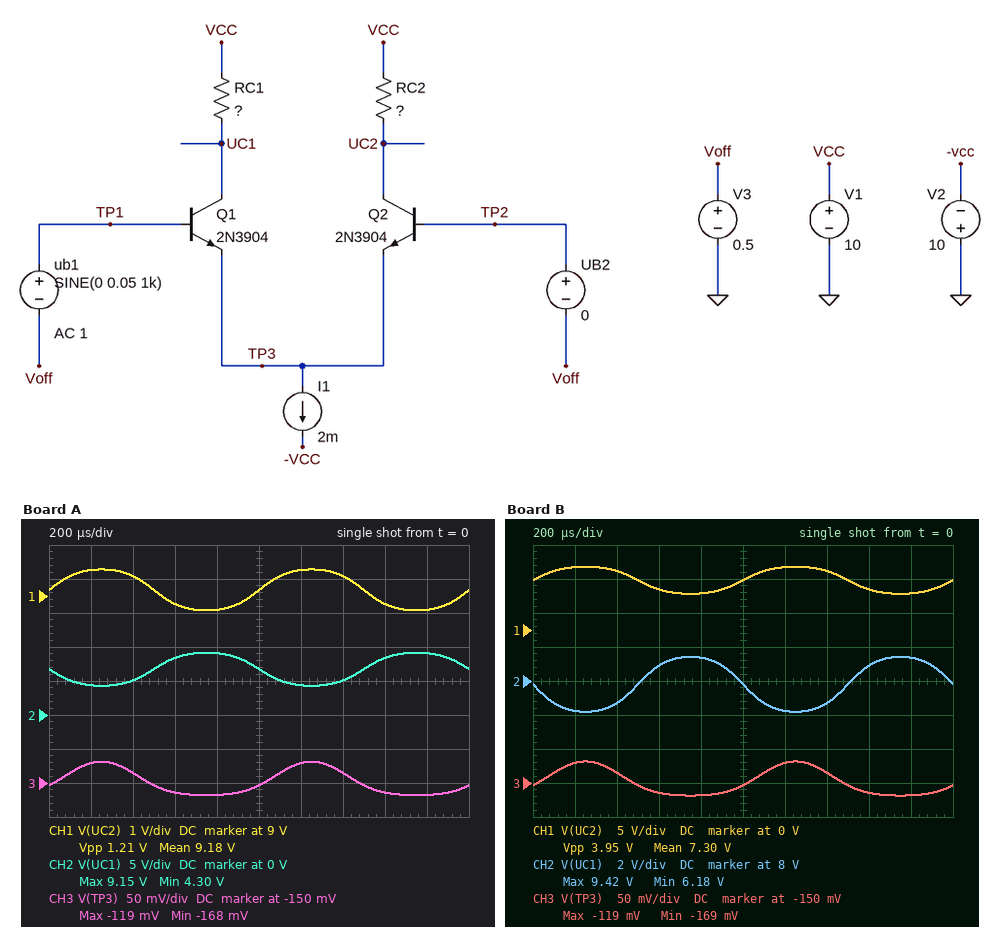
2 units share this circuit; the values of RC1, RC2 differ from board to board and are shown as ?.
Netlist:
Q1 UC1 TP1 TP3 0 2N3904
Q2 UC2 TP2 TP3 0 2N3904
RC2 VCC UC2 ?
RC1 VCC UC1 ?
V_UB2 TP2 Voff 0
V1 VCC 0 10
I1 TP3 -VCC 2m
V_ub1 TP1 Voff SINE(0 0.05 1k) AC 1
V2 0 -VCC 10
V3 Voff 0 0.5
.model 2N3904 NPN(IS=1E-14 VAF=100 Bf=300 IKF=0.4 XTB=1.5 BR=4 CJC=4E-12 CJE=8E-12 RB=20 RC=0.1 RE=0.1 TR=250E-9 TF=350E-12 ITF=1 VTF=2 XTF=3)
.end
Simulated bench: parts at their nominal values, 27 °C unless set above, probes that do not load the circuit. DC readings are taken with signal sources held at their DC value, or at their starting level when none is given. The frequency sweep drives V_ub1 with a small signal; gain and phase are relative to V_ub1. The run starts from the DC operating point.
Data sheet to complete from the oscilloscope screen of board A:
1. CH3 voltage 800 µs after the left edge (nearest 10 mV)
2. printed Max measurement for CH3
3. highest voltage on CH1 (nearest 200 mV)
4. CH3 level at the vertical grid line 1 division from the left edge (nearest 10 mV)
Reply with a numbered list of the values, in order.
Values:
1. -170 mV
2. -119 mV
3. 9.8 V
4. -120 mV
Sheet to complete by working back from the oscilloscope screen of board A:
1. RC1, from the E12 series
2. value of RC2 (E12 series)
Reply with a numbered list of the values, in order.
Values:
1. 3.3 kΩ
2. 820 Ω
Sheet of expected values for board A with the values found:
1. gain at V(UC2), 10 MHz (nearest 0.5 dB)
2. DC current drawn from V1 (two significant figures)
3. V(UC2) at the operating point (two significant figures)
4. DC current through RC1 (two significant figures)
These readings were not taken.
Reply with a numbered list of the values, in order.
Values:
1. 23.0 dB
2. 2.0 mA
3. 9.2 V
4. 990 µA
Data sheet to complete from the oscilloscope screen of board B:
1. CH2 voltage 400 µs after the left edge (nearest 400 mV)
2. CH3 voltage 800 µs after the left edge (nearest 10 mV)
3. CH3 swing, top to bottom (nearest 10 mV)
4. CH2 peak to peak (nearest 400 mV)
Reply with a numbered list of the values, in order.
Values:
1. 6.8 V
2. -170 mV
3. 50 mV
4. 3.2 V
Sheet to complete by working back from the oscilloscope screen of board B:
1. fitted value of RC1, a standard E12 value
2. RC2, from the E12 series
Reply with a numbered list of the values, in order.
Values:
1. 2.2 kΩ
2. 2.7 kΩ
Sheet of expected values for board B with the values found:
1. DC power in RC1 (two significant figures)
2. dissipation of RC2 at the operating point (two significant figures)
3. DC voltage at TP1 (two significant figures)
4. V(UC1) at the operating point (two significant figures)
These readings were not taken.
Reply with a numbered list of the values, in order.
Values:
1. 2.2 mW
2. 2.7 mW
3. 500 mV
4. 7.8 V
